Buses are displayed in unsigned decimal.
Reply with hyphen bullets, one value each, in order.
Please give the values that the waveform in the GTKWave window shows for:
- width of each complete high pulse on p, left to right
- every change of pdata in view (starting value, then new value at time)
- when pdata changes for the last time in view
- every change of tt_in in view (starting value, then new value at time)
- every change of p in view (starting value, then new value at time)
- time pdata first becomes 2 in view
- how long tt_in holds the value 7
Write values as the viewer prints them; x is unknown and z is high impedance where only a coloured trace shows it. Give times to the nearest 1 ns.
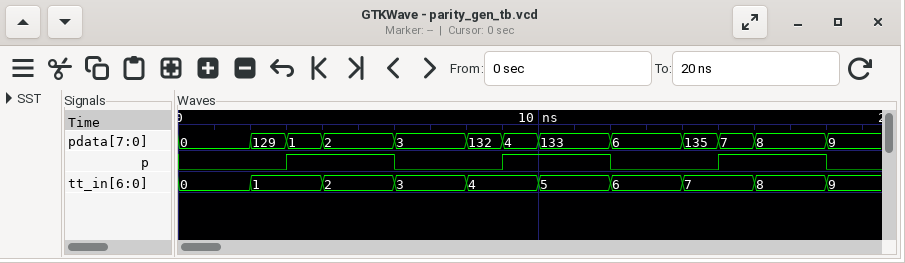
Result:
- 3 ns, 3 ns, 3 ns
- 0, 129 at 2 ns, 1 at 3 ns, 2 at 4 ns, 3 at 6 ns, 132 at 8 ns, 4 at 9 ns, 133 at 10 ns, 6 at 12 ns, 135 at 14 ns, 7 at 15 ns, 8 at 16 ns, 9 at 18 ns
- 18 ns
- 0, 1 at 2 ns, 2 at 4 ns, 3 at 6 ns, 4 at 8 ns, 5 at 10 ns, 6 at 12 ns, 7 at 14 ns, 8 at 16 ns, 9 at 18 ns
- 0, 1 at 3 ns, 0 at 6 ns, 1 at 9 ns, 0 at 12 ns, 1 at 15 ns, 0 at 18 ns
- 4 ns
- 2 ns
